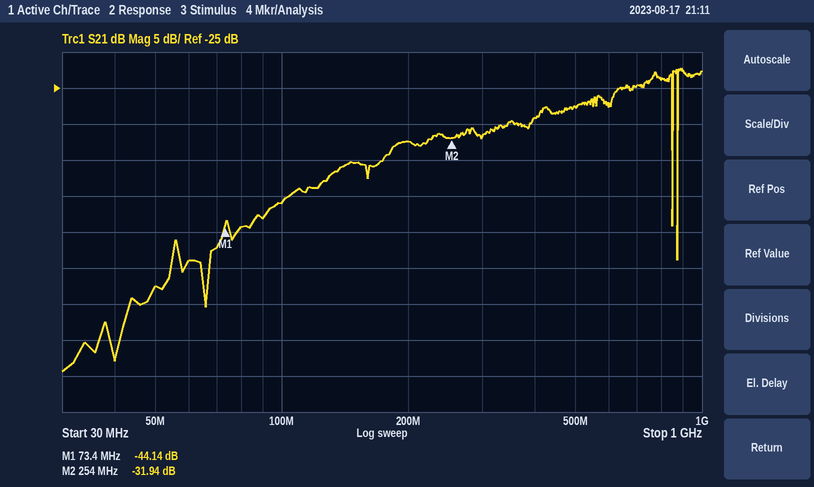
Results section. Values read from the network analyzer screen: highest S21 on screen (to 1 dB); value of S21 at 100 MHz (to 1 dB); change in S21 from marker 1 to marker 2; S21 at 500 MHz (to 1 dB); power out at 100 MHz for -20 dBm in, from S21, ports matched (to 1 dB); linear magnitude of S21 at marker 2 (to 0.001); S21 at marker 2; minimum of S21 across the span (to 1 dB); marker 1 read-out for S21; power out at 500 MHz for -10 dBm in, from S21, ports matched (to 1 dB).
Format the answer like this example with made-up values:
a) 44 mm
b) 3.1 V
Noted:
a) -22 dB
b) -41 dB
c) 12.20 dB
d) -28 dB
e) -61 dBm
f) 0.025
g) -31.94 dB
h) -64 dB
i) -44.14 dB
j) -38 dBm
